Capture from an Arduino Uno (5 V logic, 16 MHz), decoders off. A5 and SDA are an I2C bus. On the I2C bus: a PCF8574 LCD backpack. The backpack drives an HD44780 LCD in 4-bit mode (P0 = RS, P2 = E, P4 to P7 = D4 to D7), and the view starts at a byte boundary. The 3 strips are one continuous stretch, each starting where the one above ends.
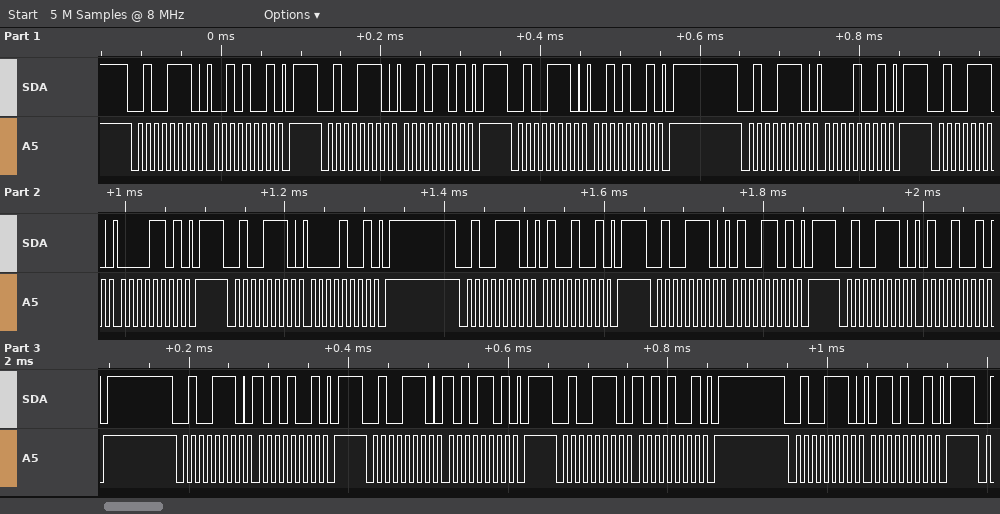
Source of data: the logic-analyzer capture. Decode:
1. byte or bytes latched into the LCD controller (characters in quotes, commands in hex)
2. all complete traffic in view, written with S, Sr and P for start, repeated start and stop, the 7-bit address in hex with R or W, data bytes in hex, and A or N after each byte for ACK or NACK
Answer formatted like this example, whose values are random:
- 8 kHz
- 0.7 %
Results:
- ' ' 'J'
- S 27W A 29 A P S 27W A 2D A P S 27W A 29 A P S 27W A 09 A P S 27W A 0D A P S 27W A 09 A P S 27W A 49 A P S 27W A 4D A P S 27W A 49 A P S 27W A A9 A P S 27W A AD A P S 27W A A9 A P S 27W A 69 A P
